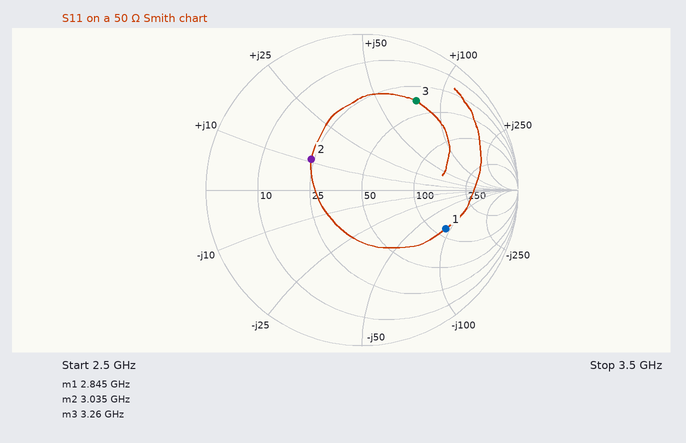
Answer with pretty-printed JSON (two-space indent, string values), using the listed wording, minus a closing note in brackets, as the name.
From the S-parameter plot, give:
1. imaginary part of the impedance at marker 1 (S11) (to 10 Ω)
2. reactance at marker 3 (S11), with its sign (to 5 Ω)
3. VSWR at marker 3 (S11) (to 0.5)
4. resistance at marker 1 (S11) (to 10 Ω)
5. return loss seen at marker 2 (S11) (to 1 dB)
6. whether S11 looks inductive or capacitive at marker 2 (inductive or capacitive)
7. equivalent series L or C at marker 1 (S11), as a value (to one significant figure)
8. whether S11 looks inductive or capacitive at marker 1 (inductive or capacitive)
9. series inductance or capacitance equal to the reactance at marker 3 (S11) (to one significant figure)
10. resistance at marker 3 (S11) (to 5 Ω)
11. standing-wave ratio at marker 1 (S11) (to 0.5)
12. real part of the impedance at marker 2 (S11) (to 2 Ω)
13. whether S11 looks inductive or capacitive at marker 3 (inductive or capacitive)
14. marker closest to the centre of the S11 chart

{
  "imaginary part of the impedance at marker 1 (S11)": "-90 Ω",
  "reactance at marker 3 (S11), with its sign": "+75 Ω",
  "VSWR at marker 3 (S11)": "5.0",
  "resistance at marker 1 (S11)": "120 Ω",
  "return loss seen at marker 2 (S11)": "8 dB",
  "whether S11 looks inductive or capacitive at marker 2": "inductive",
  "equivalent series L or C at marker 1 (S11), as a value": "600 fF",
  "whether S11 looks inductive or capacitive at marker 1": "capacitive",
  "series inductance or capacitance equal to the reactance at marker 3 (S11)": "4 nH",
  "resistance at marker 3 (S11)": "35 Ω",
  "standing-wave ratio at marker 1 (S11)": "4.0",
  "real part of the impedance at marker 2 (S11)": "24 Ω",
  "whether S11 looks inductive or capacitive at marker 3": "inductive",
  "marker closest to the centre of the S11 chart": "marker 2"
}
